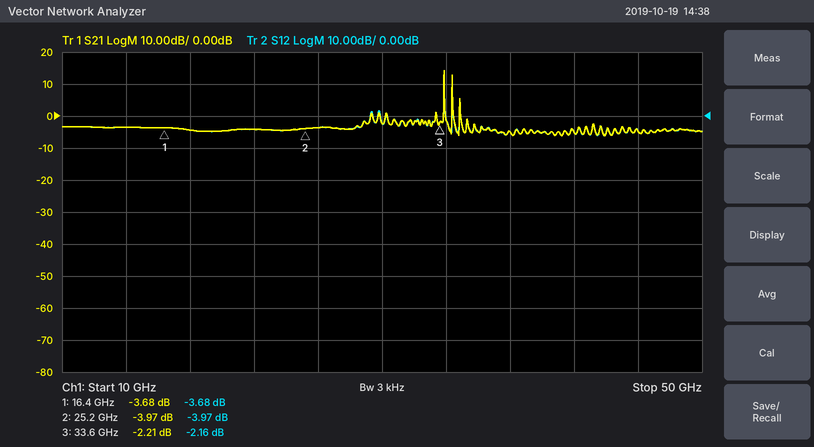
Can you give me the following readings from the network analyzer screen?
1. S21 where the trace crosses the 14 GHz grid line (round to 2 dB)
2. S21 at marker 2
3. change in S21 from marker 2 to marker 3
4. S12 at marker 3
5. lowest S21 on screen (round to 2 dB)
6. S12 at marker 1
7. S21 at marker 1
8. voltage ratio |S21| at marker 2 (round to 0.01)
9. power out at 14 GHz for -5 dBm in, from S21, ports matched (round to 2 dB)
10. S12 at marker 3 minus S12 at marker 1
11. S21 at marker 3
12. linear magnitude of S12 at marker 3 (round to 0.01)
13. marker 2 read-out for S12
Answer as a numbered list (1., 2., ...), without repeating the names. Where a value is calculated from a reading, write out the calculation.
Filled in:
1. -4 dB
2. -3.97 dB
3. -2.21 − (-3.97) = 1.76 dB
4. -2.16 dB
5. -6 dB
6. -3.68 dB
7. -3.68 dB
8. 10^(-3.97/20) ≈ 0.63
9. -5 dBm + (-4 dB) = -8 dBm
10. -2.16 − (-3.68) = 1.52 dB
11. -2.21 dB
12. 10^(-2.16/20) ≈ 0.78
13. -3.97 dB
